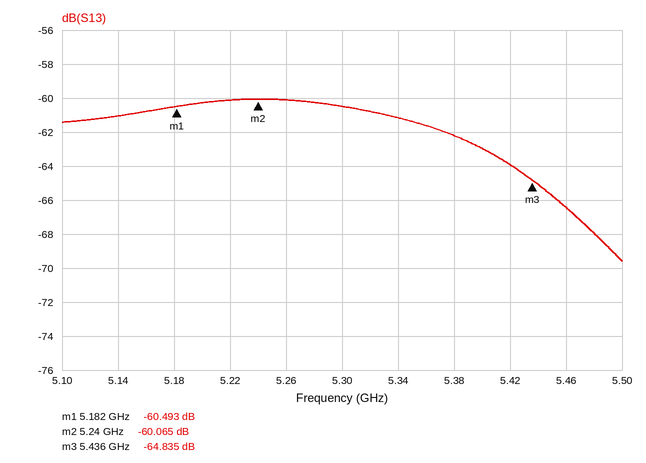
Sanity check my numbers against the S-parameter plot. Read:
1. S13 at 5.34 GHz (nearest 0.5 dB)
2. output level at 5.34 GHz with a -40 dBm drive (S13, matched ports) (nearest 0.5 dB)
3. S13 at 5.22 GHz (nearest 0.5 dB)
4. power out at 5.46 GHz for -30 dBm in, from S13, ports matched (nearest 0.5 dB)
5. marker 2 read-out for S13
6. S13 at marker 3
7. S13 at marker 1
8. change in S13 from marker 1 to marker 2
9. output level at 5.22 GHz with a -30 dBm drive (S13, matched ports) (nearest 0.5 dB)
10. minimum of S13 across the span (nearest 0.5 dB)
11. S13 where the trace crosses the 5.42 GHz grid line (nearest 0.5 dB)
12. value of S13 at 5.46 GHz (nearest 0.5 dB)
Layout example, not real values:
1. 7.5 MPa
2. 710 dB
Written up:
1. -61.0 dB
2. -101.0 dBm
3. -60.0 dB
4. -96.5 dBm
5. -60.065 dB
6. -64.835 dB
7. -60.493 dB
8. 0.428 dB
9. -90.0 dBm
10. -69.5 dB
11. -64.0 dB
12. -66.5 dB
